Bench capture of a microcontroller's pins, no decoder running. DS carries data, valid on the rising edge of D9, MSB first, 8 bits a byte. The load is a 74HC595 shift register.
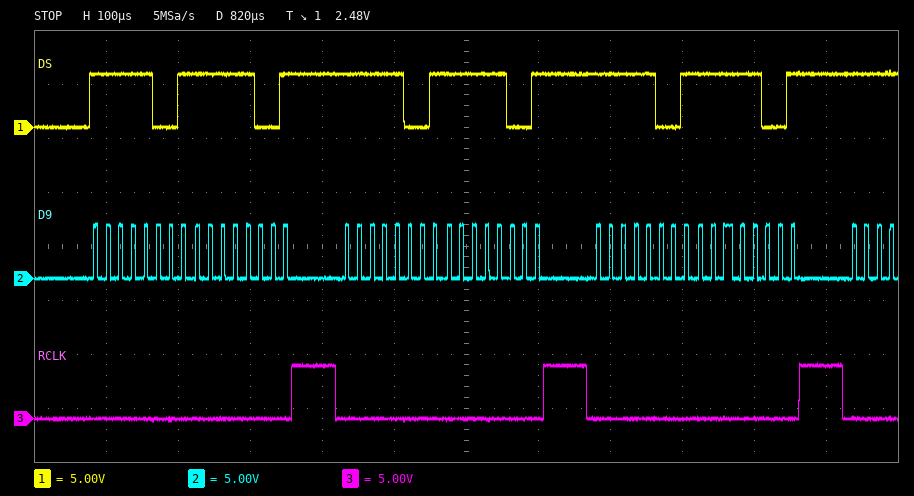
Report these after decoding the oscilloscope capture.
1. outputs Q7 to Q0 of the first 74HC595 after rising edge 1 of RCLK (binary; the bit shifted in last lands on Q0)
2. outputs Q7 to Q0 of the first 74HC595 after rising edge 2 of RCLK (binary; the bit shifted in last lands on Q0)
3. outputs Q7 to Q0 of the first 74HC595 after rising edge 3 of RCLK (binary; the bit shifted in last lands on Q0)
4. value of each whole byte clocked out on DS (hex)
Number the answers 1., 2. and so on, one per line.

1. 11111001
2. 11111001
3. 11111001
4. F9 F9 F9 F9 F9 F9
